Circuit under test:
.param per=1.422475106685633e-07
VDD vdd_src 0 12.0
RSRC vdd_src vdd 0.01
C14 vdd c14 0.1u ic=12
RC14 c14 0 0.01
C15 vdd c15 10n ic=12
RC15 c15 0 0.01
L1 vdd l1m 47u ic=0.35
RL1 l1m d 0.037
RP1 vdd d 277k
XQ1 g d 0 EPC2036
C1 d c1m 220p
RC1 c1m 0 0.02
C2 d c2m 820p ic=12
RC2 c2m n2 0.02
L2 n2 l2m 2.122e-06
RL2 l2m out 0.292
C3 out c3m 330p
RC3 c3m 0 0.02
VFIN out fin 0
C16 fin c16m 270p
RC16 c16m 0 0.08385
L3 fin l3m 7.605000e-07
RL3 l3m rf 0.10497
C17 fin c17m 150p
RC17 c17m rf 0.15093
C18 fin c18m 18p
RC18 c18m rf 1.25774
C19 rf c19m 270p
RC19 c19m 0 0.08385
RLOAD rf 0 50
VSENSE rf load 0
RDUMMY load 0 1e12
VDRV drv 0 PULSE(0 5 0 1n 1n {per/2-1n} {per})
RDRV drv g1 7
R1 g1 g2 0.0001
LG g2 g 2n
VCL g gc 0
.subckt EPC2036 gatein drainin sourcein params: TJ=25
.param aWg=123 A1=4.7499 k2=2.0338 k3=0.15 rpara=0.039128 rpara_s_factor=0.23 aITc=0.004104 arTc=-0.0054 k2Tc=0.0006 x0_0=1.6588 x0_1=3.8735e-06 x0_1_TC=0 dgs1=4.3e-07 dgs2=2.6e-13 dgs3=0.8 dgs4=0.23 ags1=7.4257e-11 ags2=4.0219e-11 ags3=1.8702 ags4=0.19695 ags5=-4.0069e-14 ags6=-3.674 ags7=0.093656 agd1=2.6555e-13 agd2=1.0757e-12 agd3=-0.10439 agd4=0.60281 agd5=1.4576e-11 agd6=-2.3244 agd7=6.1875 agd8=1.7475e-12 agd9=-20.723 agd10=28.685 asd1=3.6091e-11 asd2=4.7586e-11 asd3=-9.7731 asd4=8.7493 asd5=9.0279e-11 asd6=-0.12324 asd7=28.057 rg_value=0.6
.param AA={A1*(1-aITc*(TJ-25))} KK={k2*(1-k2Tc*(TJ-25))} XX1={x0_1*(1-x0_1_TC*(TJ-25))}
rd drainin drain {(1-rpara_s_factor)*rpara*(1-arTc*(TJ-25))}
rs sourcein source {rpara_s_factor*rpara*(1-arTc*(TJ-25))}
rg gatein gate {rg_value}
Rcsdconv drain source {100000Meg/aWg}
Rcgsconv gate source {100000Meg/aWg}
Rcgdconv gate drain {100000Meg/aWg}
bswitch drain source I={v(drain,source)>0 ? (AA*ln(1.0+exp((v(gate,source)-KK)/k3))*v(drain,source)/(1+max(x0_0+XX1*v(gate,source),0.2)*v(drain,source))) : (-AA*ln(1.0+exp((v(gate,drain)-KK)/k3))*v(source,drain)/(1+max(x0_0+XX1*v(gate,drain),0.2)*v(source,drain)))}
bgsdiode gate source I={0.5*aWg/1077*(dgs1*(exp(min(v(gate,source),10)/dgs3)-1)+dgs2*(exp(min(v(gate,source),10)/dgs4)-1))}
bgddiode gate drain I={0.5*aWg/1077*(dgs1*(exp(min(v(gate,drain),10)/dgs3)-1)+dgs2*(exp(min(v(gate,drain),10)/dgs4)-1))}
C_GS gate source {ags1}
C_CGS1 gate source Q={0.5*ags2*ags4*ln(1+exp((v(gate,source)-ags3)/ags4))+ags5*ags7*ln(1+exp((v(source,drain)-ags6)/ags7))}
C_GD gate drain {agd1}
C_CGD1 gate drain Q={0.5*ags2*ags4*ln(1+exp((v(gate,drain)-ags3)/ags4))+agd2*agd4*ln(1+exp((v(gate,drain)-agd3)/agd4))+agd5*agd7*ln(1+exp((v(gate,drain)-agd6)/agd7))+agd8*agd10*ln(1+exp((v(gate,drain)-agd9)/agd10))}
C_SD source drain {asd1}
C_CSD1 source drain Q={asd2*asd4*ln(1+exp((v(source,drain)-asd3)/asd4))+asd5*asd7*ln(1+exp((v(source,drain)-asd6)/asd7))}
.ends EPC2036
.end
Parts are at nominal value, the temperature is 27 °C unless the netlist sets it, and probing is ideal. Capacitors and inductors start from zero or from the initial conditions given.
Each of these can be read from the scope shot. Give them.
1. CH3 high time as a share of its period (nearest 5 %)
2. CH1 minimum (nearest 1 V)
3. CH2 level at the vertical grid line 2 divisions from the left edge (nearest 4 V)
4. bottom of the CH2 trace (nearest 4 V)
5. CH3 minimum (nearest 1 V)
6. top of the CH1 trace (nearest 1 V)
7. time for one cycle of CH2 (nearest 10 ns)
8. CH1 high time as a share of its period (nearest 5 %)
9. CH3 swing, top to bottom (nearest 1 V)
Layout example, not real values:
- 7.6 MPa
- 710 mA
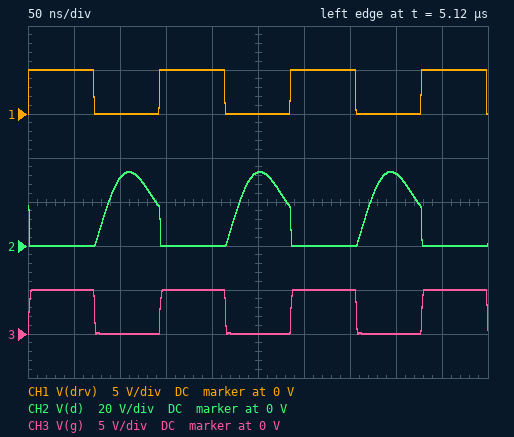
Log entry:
- 50 %
- 0 V
- 32 V
- 0 V
- 0 V
- 5 V
- 140 ns
- 50 %
- 5 V
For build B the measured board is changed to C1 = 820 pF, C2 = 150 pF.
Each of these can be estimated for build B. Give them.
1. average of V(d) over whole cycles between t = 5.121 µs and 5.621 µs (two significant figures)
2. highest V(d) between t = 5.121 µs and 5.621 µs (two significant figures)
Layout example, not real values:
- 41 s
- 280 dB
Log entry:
- 11 V
- 47 V
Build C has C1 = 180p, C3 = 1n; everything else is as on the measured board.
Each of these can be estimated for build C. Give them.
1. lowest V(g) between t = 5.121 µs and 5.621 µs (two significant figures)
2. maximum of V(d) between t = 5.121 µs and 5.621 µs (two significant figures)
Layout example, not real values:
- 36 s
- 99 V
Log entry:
- -67 mV
- 40 V
